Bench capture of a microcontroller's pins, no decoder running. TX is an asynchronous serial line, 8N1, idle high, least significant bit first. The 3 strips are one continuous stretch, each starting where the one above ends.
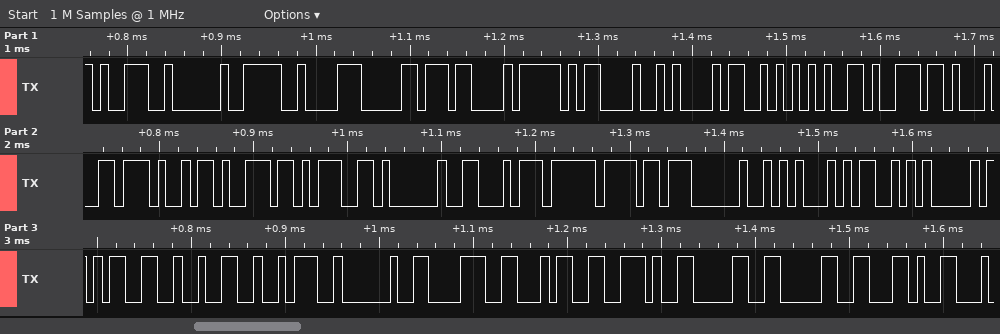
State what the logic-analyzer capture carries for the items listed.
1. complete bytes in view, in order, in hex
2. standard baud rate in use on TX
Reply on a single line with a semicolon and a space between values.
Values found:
39 20 C2 B0 43 0D 0A 53 65 6E 64 69 6E 67 20 74 6F 20 45 53 50 33 32 3A 20 38 34 2E 30 30 2C; 115200 baud
